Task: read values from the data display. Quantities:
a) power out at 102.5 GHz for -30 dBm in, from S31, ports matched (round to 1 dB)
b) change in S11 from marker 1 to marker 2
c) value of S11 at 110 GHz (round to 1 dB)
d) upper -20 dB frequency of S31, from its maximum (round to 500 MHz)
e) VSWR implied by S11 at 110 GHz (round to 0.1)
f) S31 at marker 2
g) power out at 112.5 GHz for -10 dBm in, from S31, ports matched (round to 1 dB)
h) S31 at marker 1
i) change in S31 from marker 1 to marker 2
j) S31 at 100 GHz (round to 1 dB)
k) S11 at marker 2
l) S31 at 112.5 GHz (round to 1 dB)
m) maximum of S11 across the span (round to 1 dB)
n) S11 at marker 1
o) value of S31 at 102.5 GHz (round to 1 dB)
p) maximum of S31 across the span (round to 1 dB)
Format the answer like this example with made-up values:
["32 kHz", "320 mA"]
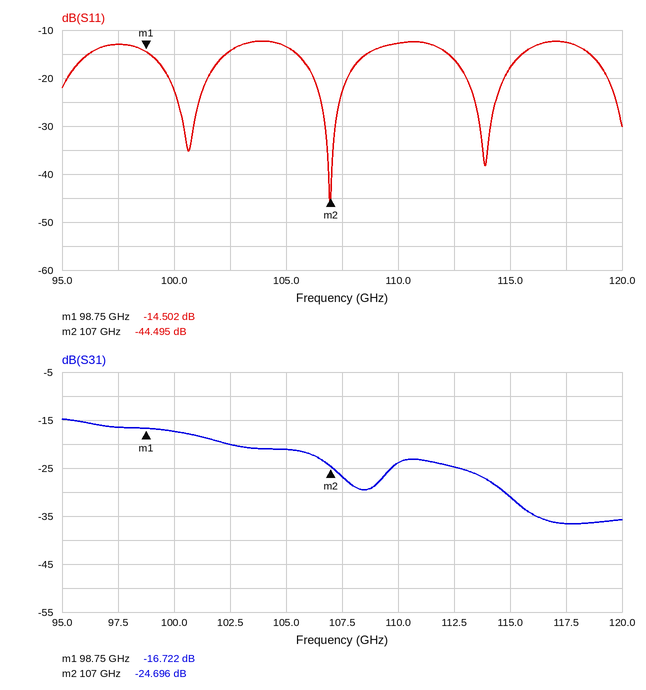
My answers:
["-50 dBm", "-29.993 dB", "-13 dB", "116.0 GHz", "1.6", "-24.696 dB", "-35 dBm", "-16.722 dB", "-7.974 dB", "-17 dB", "-44.495 dB", "-25 dB", "-12 dB", "-14.502 dB", "-20 dB", "-15 dB"]
